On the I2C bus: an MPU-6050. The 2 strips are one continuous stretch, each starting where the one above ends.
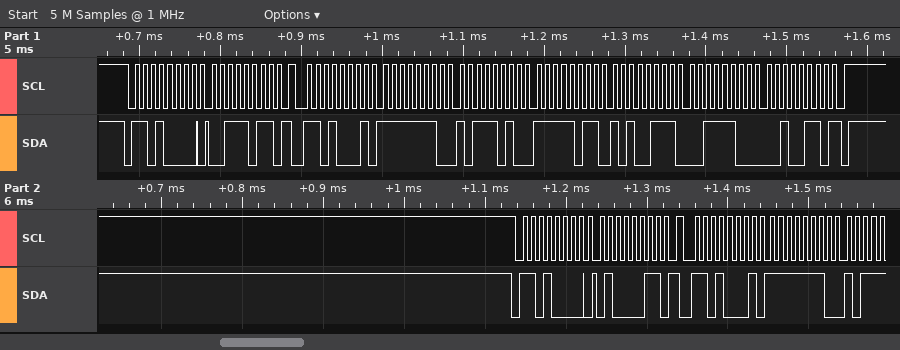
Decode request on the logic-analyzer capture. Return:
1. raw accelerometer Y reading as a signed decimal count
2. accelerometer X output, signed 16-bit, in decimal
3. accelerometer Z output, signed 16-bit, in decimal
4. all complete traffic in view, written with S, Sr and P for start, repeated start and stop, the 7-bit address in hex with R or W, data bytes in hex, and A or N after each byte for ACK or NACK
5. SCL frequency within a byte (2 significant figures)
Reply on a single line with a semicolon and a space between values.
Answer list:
-1113; -326; 15398; S 68W A 3B A Sr 68R A FE A BA A FB A A7 A 3C A 26 N P S 68W A 43 A Sr 68R A FE A; 100 kHz
